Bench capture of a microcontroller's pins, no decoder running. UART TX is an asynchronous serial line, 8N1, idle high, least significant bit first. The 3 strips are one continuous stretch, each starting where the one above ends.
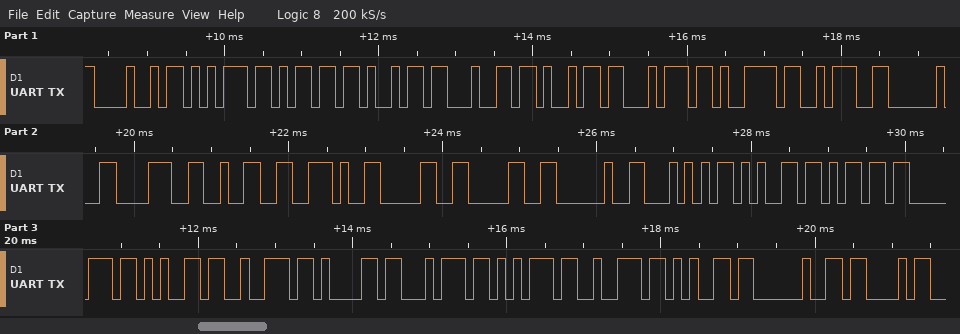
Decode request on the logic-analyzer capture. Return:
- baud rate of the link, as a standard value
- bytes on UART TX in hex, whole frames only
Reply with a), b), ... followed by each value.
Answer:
a) 9600 baud
b) 48 75 6D 69 64 69 74 79 3A 20 38 32 2E 30 30 20 54 65 6D 70 65 72 61 74 75 72 65 20 43
